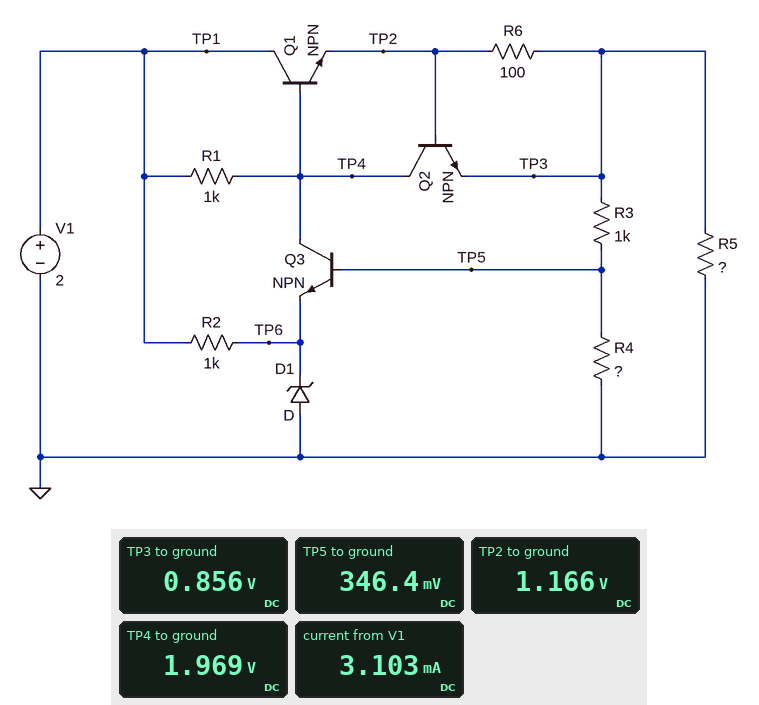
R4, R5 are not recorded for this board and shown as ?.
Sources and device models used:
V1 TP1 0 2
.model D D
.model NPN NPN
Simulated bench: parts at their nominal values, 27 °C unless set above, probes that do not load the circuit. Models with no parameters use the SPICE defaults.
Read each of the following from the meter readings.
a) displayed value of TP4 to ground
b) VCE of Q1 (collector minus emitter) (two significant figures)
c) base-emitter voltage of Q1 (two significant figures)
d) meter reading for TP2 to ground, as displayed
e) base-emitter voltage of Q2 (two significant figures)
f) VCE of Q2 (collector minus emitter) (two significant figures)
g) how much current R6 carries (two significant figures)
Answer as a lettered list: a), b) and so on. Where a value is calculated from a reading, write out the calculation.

a) 1.969 V
b) 2 V - 1.166 V = 830 mV
c) 1.969 V - 1.166 V = 800 mV
d) 1.166 V
e) 1.166 V - 856 mV = 310 mV
f) 1.969 V - 856 mV = 1.1 V
g) (1.166 V - 856 mV) / 100 Ω = 3.1 mA
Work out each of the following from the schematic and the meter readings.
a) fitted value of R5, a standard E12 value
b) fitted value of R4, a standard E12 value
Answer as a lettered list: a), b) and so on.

a) 330 Ω
b) 680 Ω
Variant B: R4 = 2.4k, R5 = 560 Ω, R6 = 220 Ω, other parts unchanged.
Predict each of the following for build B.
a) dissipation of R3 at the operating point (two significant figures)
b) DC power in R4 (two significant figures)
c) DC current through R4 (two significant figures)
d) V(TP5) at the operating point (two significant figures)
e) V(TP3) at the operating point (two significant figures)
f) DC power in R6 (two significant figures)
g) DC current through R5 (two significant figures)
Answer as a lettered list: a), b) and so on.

a) 58 µW
b) 140 µW
c) 240 µA
d) 580 mV
e) 820 mV
f) 640 µW
g) 1.5 mA
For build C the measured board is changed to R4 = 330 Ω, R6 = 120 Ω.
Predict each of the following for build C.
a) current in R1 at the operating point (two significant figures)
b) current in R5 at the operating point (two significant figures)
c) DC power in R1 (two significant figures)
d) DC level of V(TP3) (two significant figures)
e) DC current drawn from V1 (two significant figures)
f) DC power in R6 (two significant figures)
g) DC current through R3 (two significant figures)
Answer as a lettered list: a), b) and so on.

a) 30 µA
b) 2.4 mA
c) 900 nW
d) 800 mV
e) 3.0 mA
f) 1.1 mW
g) 600 µA
